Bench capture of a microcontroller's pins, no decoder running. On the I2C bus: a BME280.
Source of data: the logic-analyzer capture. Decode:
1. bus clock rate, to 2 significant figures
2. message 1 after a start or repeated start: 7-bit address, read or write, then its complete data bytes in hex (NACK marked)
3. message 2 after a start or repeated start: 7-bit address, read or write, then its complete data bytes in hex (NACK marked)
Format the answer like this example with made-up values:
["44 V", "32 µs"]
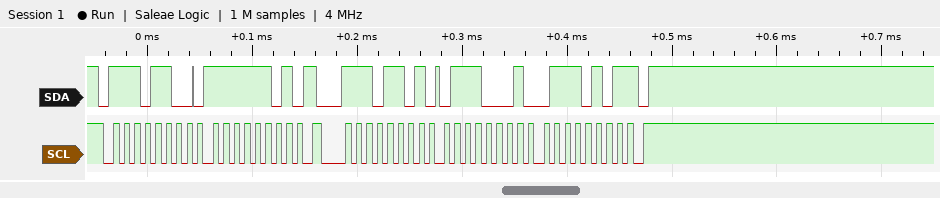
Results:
["100 kHz", "0x76 write: FD", "0x76 read: 71 75 NACK"]
